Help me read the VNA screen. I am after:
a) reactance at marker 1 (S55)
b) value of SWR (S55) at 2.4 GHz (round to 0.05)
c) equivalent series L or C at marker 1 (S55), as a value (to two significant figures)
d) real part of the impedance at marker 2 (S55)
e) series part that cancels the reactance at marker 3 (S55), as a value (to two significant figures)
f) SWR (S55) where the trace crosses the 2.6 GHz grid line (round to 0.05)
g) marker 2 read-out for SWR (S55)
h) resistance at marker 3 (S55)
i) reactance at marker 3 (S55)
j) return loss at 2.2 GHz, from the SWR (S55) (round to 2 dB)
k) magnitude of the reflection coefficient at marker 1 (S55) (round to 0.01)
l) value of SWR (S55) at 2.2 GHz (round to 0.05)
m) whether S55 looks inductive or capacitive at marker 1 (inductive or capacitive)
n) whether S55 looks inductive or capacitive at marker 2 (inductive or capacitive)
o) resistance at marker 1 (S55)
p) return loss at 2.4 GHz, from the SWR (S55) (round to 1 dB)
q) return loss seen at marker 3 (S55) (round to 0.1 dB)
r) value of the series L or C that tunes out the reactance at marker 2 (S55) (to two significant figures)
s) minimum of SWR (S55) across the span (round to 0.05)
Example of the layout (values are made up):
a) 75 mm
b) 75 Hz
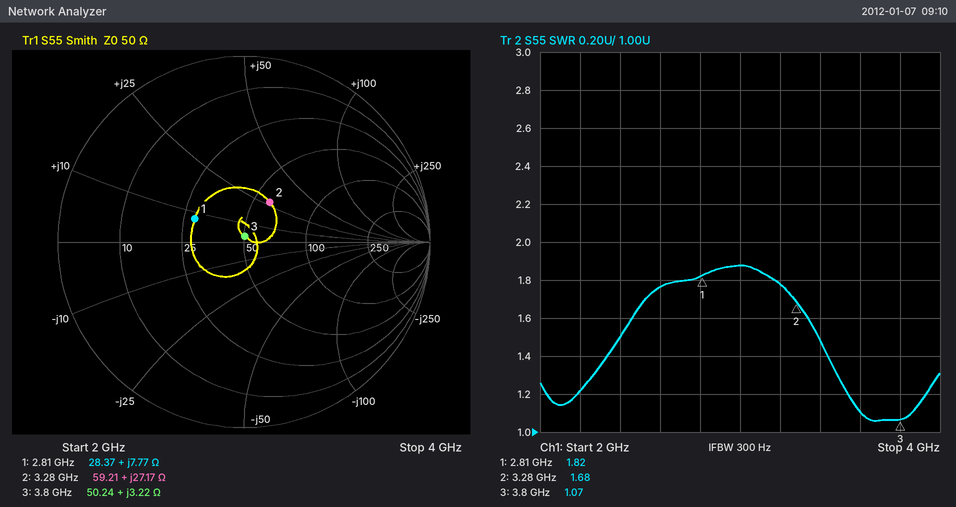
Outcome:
a) +7.77 Ω
b) 1.50
c) 440 pH
d) 59.21 Ω
e) 13 pF
f) 1.75
g) 1.68
h) 50.24 Ω
i) +3.22 Ω
j) 20 dB
k) 0.29
l) 1.20
m) inductive
n) inductive
o) 28.37 Ω
p) 14 dB
q) 29.8 dB
r) 1.8 pF
s) 1.05
